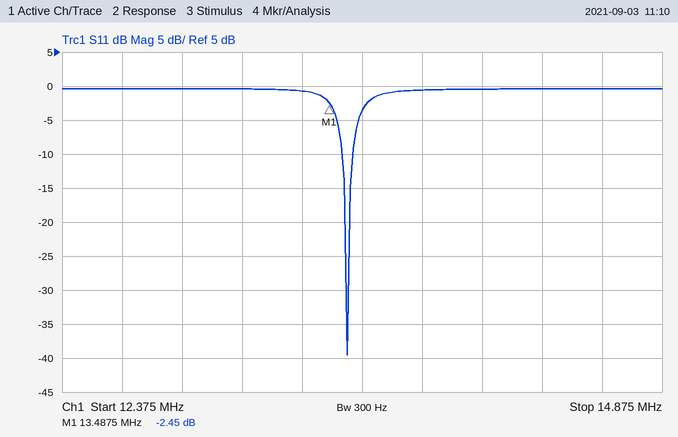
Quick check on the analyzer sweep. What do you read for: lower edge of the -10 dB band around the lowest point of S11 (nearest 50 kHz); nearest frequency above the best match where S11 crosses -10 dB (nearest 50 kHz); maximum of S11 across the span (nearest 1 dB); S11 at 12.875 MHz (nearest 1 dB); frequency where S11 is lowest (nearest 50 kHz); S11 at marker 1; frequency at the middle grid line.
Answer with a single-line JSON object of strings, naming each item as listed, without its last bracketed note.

{"lower edge of the -10 dB band around the lowest point of S11": "13.55 MHz", "nearest frequency above the best match where S11 crosses -10 dB": "13.60 MHz", "maximum of S11 across the span": "0 dB", "S11 at 12.875 MHz": "0 dB", "frequency where S11 is lowest": "13.55 MHz", "S11 at marker 1": "-2.45 dB", "frequency at the middle grid line": "13.625 MHz"}
